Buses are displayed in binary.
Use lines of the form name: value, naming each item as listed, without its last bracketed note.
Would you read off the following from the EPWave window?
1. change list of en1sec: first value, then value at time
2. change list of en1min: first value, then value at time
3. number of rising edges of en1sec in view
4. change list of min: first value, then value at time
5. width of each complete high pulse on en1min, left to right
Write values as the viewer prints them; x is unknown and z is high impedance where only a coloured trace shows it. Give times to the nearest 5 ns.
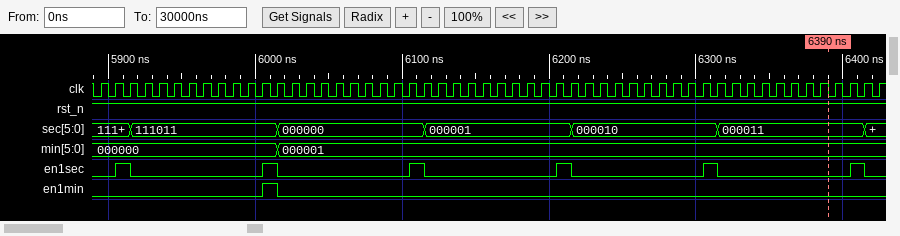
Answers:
change list of en1sec: first value, then value at time: 0, 1 at 5905 ns, 0 at 5915 ns, 1 at 6005 ns, 0 at 6015 ns, 1 at 6105 ns, 0 at 6115 ns, 1 at 6205 ns, 0 at 6215 ns, 1 at 6305 ns, 0 at 6315 ns, 1 at 6405 ns, 0 at 6415 ns
change list of en1min: first value, then value at time: 0, 1 at 6005 ns, 0 at 6015 ns
number of rising edges of en1sec in view: 6
change list of min: first value, then value at time: 000000, 000001 at 6015 ns
width of each complete high pulse on en1min, left to right: 10 ns
